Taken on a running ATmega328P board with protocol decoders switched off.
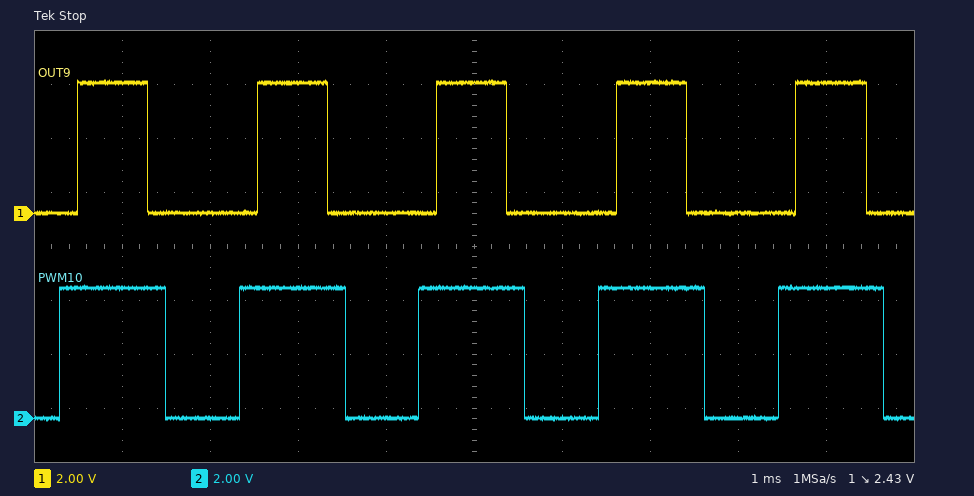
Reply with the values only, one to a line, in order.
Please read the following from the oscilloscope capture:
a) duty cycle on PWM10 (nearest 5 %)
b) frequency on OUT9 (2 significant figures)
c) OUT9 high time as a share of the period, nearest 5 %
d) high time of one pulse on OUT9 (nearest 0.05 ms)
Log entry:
60 %
490 Hz
40 %
0.80 ms
